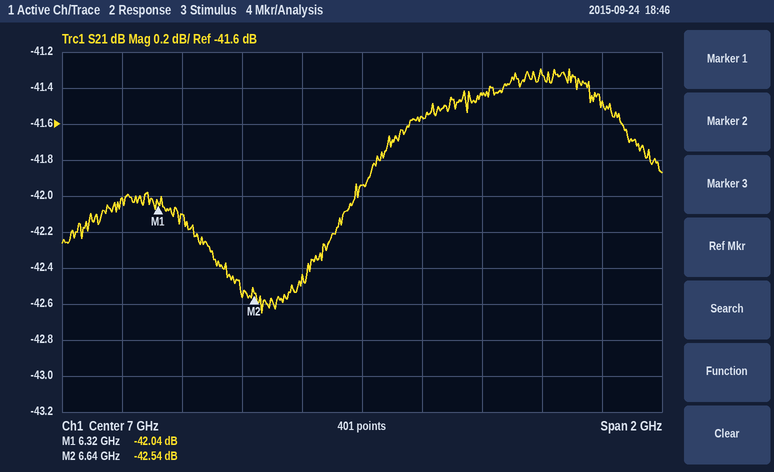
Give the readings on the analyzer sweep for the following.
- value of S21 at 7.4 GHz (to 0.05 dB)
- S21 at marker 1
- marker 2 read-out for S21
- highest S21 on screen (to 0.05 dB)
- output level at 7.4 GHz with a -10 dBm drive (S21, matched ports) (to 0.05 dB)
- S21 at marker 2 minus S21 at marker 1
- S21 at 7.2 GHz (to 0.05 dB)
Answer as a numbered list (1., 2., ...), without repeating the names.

1. -41.45 dB
2. -42.04 dB
3. -42.54 dB
4. -41.30 dB
5. -51.45 dBm
6. -0.50 dB
7. -41.55 dB
